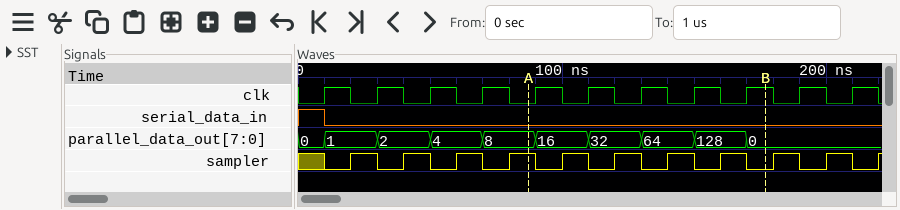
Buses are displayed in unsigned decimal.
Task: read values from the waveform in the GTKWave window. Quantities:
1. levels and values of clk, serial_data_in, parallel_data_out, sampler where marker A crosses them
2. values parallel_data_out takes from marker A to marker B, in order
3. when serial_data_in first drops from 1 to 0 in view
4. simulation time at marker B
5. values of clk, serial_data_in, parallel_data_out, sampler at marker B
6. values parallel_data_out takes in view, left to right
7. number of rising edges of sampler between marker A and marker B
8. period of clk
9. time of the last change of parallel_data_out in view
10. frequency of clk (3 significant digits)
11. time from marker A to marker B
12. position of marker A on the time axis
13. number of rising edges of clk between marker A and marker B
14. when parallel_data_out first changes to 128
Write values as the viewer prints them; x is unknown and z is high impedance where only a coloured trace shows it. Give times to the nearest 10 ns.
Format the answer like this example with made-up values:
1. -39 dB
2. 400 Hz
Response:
1. clk=0, serial_data_in=0, parallel_data_out=8, sampler=1
2. 8, 16, 32, 64, 128, 0
3. 10 ns
4. 180 ns
5. clk=1, serial_data_in=0, parallel_data_out=0, sampler=0
6. 0, 1, 2, 4, 8, 16, 32, 64, 128, 0
7. 4
8. 20 ns
9. 170 ns
10. 50.0 MHz
11. 90 ns
12. 90 ns
13. 5
14. 150 ns
